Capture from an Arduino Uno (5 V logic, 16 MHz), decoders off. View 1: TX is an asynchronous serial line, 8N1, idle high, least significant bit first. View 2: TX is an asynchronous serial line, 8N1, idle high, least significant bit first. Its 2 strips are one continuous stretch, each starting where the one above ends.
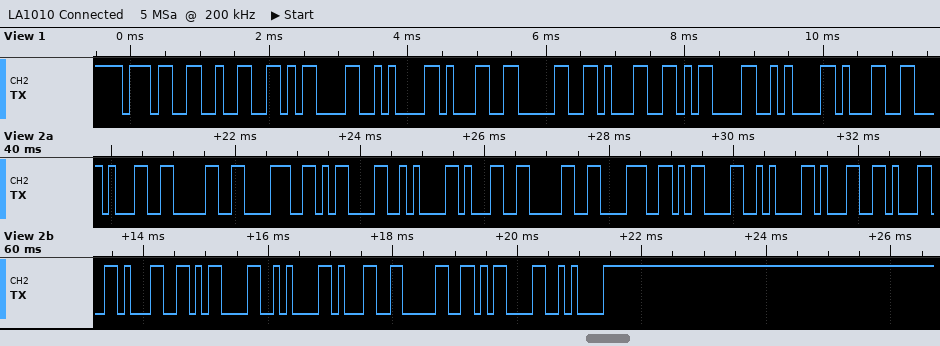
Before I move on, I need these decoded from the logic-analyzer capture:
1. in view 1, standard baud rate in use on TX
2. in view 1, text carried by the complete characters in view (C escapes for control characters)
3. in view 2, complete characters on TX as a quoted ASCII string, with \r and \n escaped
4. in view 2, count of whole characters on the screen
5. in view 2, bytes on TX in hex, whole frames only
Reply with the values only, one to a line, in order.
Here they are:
9600 baud
"72\r\n101\r\n1"
"108\r\n108\r\n111\r\n10\r\n"
19
0x31 0x30 0x38 0x0D 0x0A 0x31 0x30 0x38 0x0D 0x0A 0x31 0x31 0x31 0x0D 0x0A 0x31 0x30 0x0D 0x0A
